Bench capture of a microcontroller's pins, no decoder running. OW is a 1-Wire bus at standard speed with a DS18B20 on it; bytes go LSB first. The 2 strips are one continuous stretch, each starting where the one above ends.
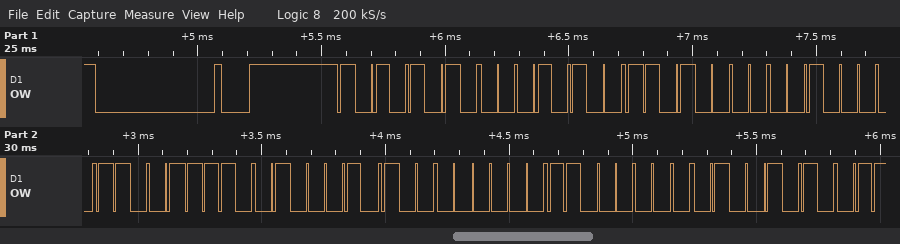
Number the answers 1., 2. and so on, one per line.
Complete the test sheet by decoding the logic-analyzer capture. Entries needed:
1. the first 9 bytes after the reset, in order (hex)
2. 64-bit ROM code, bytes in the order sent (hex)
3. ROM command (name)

1. 55 28 0B 84 79 A2 00 03 52
2. 28 0B 84 79 A2 00 03 52
3. Match ROM
